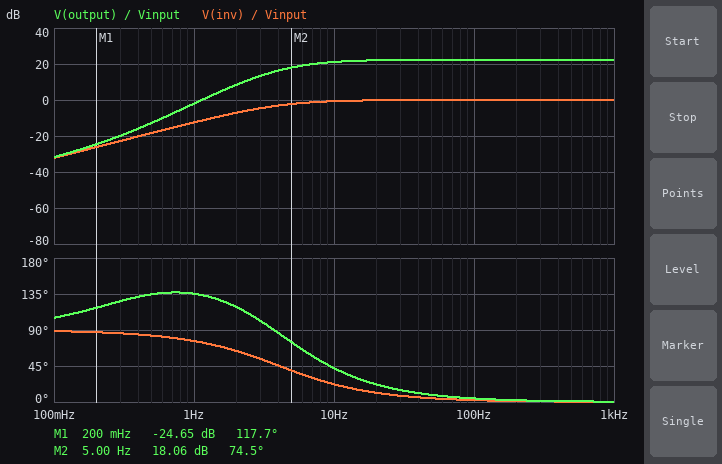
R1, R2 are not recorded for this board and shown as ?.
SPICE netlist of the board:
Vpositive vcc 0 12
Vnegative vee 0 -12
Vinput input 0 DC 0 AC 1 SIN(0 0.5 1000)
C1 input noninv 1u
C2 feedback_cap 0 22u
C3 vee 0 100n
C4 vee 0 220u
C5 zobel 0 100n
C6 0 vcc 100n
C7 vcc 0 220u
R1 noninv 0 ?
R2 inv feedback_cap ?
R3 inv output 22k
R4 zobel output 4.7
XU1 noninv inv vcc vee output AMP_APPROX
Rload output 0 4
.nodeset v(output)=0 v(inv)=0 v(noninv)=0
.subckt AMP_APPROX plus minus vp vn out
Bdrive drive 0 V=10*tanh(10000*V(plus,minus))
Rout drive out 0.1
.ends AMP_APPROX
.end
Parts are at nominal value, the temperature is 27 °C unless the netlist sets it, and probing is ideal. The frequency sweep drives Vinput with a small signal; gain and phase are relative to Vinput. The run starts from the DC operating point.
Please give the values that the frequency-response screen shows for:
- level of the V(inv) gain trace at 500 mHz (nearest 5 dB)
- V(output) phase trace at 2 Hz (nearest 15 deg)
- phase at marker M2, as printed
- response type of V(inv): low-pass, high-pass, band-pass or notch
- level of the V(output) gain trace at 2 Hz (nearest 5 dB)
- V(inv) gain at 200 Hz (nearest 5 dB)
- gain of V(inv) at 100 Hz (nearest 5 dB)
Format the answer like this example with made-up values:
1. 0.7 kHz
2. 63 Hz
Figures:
1. -20 dB
2. 120 deg
3. 74.5 deg
4. high-pass
5. 10 dB
6. 0 dB
7. 0 dB
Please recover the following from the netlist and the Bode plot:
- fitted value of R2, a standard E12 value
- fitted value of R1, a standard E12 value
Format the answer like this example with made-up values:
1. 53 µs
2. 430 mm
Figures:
1. 1.8 kΩ
2. 39 kΩ
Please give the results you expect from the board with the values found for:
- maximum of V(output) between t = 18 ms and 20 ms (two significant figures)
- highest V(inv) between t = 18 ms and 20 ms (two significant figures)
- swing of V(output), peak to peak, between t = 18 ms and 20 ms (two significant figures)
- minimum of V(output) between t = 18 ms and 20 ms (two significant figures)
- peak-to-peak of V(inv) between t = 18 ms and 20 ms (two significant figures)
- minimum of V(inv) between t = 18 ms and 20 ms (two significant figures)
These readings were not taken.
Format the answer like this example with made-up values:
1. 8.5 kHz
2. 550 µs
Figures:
1. 6.6 V
2. 500 mV
3. 13 V
4. -6.6 V
5. 1.0 V
6. -500 mV
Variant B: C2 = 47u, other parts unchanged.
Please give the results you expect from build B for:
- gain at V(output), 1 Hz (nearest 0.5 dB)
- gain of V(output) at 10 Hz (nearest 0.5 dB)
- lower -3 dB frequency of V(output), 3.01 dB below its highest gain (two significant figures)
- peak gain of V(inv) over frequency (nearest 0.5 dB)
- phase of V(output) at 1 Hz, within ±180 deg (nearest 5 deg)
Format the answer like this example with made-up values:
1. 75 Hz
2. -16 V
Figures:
1. 3.5 dB
2. 21.5 dB
3. 4.8 Hz
4. 0 dB
5. 130 deg
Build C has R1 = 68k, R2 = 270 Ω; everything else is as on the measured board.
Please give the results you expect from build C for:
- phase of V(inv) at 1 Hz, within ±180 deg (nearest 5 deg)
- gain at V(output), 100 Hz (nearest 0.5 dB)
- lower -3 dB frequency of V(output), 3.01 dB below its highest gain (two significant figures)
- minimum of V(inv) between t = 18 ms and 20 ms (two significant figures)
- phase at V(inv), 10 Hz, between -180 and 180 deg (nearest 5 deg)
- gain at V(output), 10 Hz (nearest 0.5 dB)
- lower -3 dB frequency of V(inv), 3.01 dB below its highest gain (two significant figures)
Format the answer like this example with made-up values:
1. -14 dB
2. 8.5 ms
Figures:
1. 65 deg
2. 38.0 dB
3. 27 Hz
4. -120 mV
5. 15 deg
6. 29.0 dB
7. 2.3 Hz
